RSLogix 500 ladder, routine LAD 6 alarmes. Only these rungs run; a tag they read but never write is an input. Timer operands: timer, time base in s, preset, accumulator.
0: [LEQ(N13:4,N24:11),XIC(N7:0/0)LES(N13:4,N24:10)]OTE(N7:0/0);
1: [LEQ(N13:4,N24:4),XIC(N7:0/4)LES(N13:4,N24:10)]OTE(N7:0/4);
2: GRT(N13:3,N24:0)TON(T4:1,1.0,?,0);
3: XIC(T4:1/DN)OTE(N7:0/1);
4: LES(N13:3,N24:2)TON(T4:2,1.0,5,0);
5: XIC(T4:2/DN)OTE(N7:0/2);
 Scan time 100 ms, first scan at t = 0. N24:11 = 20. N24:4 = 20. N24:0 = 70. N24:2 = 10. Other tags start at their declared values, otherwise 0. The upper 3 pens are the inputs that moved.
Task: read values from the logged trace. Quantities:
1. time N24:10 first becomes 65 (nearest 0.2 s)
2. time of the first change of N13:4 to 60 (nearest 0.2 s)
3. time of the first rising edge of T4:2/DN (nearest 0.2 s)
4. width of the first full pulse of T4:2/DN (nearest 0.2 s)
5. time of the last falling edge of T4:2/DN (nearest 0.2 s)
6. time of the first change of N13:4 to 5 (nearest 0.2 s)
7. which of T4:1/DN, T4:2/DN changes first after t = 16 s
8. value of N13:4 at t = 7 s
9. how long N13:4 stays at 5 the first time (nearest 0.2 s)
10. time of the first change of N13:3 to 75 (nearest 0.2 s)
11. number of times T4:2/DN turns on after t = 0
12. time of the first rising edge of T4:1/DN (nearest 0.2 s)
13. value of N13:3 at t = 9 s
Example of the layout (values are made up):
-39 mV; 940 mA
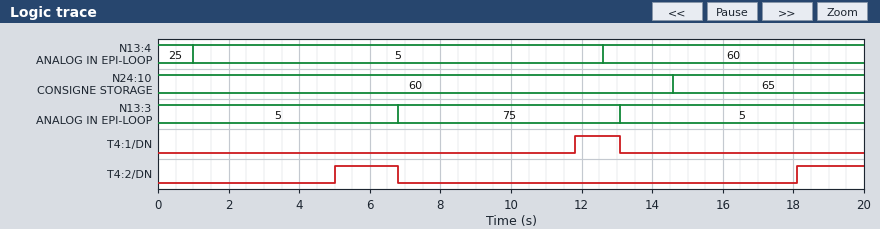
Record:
14.6 s; 12.6 s; 5.0 s; 1.8 s; 6.8 s; 1.0 s; T4:2/DN; 5; 11.6 s; 6.8 s; 2; 11.8 s; 75
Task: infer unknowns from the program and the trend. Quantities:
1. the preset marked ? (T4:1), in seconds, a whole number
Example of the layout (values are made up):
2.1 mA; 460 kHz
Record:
5 s
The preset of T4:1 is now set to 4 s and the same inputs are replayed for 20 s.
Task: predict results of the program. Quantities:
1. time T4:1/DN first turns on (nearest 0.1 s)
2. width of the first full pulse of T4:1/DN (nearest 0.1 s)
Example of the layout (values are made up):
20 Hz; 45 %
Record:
10.8 s; 2.3 s
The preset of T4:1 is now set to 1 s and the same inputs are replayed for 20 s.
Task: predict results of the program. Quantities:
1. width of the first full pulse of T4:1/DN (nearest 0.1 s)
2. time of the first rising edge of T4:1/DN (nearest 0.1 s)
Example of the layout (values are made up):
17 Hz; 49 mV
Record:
5.3 s; 7.8 s
